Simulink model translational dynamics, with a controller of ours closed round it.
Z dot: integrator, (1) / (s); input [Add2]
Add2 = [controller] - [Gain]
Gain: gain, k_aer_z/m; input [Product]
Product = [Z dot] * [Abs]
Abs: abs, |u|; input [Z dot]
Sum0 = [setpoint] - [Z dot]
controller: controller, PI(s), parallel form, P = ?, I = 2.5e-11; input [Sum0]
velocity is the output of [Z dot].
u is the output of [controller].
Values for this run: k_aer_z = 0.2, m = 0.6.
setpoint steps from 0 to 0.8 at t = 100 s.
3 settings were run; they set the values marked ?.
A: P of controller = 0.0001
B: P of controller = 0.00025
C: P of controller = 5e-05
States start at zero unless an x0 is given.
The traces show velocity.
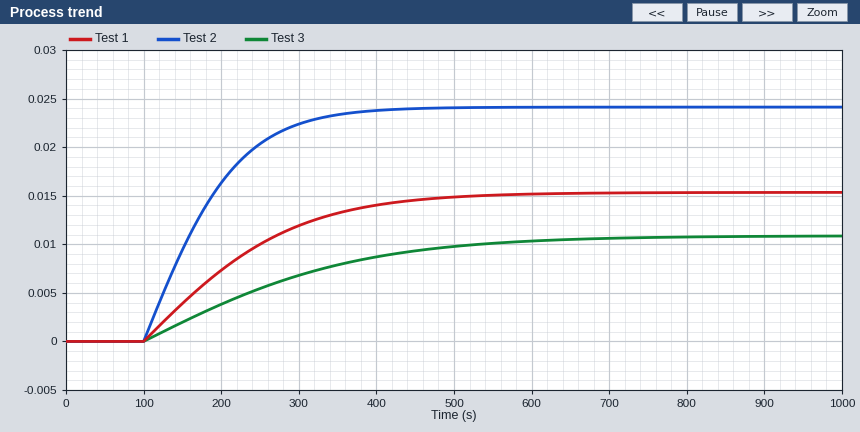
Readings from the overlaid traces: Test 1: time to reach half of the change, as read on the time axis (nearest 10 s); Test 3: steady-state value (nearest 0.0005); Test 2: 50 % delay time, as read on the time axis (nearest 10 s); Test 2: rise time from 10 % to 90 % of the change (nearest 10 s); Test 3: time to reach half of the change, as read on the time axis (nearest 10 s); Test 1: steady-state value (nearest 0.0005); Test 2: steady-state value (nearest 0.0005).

210 s
0.0110
170 s
170 s
250 s
0.0155
0.0240
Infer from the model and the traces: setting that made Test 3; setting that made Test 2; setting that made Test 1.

C
B
A
